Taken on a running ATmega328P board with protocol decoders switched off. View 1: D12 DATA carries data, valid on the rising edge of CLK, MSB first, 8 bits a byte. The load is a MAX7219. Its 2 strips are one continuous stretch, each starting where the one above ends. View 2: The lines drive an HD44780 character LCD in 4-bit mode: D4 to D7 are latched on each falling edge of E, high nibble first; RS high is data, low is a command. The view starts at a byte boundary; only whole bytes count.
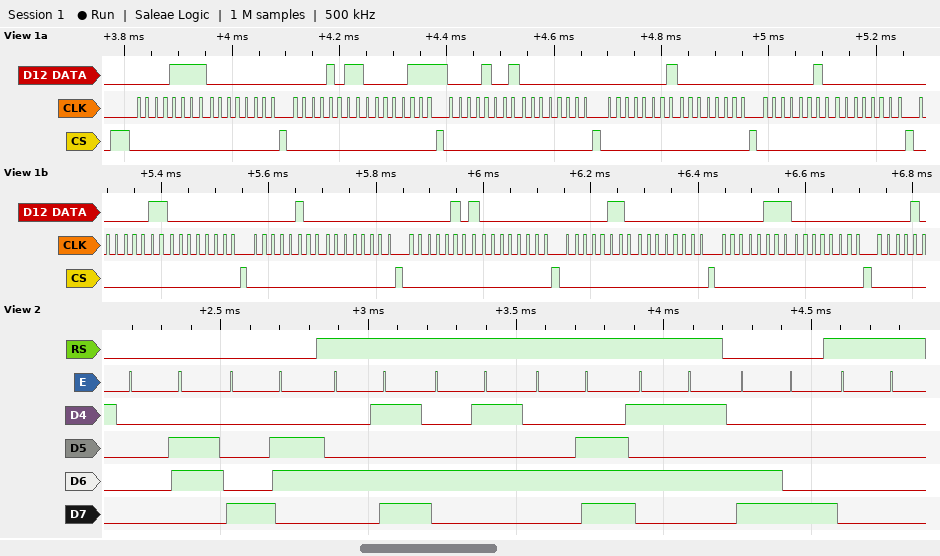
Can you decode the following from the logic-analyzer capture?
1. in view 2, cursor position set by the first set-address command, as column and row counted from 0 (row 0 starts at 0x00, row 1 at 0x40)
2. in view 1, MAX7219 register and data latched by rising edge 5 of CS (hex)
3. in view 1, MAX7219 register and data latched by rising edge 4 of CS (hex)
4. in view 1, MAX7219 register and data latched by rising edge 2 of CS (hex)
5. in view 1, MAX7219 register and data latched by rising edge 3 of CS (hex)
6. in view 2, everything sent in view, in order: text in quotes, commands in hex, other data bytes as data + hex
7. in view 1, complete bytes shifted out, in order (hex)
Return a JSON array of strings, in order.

["column 6, row 0", "register 0x1, data 0x00", "register 0x9, data 0x00", "register 0xF, data 0x00", "register 0xB, data 0x07", "0x06 0x86 \"MENU\" 0xC8 data 00", "0x0F 0x00 0x0B 0x07 0x09 0x00 0x01 0x00 0x02 0x00 0x03 0x00 0x04 0x00 0x05 0x00 0x06 0x00 0x07 0x00"]
